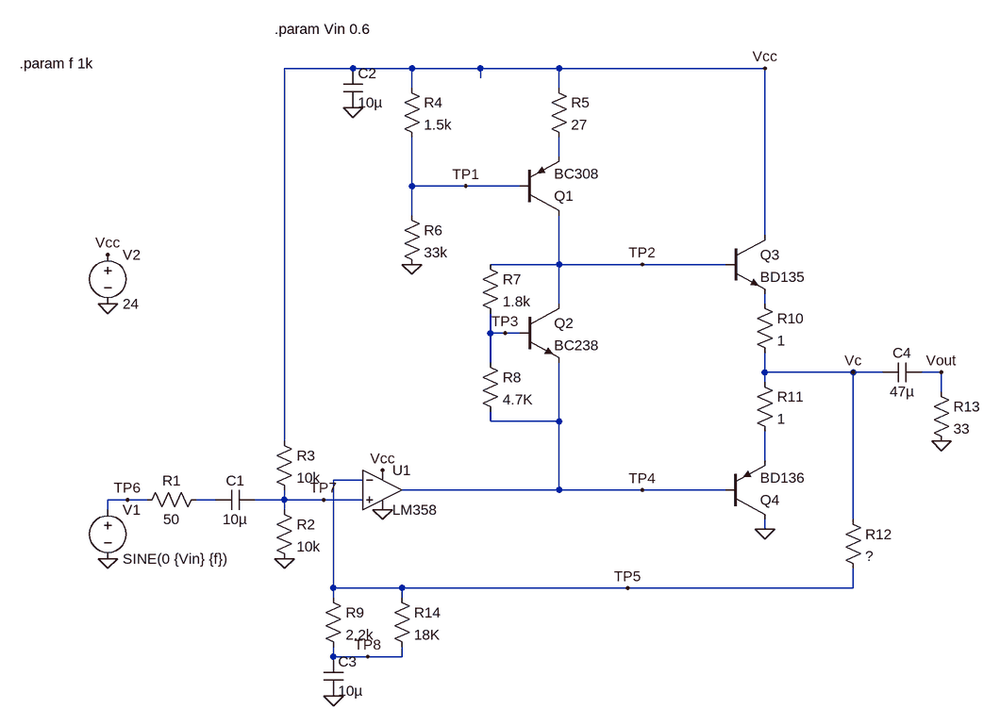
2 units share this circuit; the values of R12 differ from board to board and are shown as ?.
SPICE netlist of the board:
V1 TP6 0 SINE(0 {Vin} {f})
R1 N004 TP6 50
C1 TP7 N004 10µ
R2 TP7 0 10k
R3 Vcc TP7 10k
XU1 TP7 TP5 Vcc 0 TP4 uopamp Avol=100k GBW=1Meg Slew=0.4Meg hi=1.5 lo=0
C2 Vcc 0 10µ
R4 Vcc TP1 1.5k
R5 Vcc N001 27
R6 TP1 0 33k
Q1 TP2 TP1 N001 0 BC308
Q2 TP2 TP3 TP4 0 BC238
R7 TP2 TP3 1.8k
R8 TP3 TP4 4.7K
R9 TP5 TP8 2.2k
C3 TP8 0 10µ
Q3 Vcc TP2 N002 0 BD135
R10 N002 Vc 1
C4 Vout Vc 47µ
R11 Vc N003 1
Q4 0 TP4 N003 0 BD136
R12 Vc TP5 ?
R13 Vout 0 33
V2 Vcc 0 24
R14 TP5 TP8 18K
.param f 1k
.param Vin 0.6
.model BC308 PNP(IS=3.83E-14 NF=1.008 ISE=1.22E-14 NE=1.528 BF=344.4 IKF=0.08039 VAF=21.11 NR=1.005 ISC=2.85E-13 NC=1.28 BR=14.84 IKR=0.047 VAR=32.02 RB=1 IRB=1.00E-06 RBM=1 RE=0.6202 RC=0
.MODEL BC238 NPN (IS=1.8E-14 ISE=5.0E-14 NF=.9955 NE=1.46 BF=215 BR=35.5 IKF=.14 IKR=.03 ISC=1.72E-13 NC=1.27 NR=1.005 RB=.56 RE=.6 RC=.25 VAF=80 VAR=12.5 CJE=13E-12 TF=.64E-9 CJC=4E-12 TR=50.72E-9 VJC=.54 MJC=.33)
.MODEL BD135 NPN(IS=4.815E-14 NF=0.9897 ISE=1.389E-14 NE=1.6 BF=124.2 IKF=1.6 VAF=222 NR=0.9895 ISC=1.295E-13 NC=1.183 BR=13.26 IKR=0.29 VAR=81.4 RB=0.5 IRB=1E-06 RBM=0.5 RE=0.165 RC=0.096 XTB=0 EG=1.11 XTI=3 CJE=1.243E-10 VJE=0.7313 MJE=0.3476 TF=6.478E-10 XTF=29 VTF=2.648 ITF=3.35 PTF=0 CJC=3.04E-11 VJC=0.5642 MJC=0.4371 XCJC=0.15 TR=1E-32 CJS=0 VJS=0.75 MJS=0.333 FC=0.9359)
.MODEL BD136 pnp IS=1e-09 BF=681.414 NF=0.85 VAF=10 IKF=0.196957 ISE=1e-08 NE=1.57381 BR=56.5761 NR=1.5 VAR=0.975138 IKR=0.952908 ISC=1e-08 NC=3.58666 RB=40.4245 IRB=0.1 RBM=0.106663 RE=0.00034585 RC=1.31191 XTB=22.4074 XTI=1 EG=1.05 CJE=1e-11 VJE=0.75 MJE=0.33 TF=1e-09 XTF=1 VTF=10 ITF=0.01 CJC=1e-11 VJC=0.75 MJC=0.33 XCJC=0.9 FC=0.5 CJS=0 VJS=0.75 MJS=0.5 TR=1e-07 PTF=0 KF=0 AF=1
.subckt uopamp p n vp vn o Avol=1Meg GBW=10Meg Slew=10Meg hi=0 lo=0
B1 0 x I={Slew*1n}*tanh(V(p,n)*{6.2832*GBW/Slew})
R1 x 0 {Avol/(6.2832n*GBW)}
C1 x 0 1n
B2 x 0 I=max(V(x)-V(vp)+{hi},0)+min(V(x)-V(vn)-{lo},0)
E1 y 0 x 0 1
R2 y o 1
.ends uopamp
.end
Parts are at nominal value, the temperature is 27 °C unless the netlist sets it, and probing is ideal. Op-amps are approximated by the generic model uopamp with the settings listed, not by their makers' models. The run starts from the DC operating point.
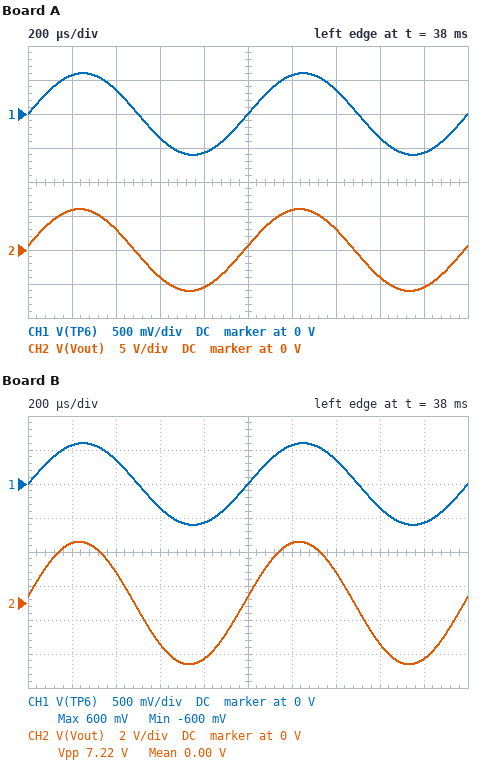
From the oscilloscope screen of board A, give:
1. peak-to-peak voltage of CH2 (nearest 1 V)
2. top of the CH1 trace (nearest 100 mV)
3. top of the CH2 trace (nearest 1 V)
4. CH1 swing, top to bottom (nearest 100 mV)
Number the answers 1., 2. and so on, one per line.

1. 12 V
2. 600 mV
3. 6 V
4. 1.2 V
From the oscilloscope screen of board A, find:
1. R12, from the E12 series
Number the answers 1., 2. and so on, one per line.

1. 18 kΩ
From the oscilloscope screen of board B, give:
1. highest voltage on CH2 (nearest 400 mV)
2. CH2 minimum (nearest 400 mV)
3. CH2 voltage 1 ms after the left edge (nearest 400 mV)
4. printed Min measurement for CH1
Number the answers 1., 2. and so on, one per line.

1. 3.6 V
2. -3.6 V
3. 400 mV
4. -600 mV
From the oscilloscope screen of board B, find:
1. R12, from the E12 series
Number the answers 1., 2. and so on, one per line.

1. 10 kΩ
